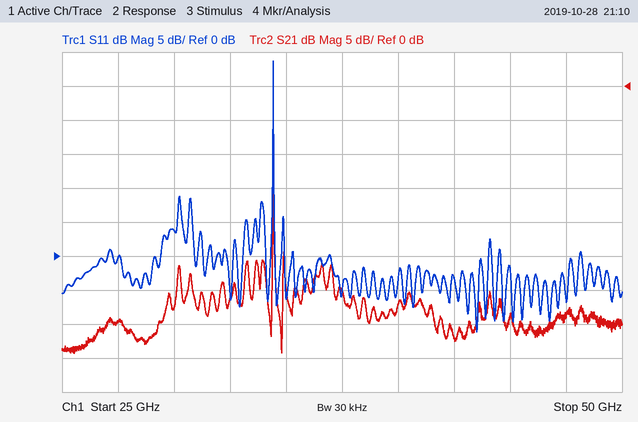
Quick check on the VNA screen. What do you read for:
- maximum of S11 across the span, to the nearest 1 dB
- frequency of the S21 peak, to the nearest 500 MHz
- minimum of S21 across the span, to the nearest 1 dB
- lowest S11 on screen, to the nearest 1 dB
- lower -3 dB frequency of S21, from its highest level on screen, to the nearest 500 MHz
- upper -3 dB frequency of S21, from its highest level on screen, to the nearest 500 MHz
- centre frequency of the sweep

29 dB
34.5 GHz
-39 dB
-11 dB
34.5 GHz
34.5 GHz
37.5 GHz
